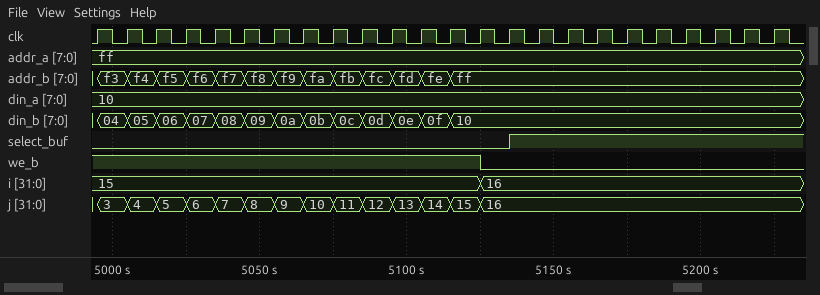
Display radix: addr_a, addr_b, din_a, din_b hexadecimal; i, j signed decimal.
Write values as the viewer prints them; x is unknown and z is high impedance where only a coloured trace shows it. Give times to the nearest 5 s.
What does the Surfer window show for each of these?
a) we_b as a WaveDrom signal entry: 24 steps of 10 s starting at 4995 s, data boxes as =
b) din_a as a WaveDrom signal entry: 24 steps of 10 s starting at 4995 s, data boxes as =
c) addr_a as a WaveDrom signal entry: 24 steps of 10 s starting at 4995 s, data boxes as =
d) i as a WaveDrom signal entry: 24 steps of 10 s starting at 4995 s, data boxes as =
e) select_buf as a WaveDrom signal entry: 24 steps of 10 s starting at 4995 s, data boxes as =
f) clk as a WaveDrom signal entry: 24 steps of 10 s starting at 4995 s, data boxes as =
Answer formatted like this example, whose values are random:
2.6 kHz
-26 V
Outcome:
{name: 'we_b', wave: '1............0..........'}
{name: 'din_a', wave: '=.......................', data: '10'}
{name: 'addr_a', wave: '=.......................', data: 'ff'}
{name: 'i', wave: '=............=..........', data: '15 16'}
{name: 'select_buf', wave: '0.............1.........'}
{name: 'clk', wave: 'p.......................'}
